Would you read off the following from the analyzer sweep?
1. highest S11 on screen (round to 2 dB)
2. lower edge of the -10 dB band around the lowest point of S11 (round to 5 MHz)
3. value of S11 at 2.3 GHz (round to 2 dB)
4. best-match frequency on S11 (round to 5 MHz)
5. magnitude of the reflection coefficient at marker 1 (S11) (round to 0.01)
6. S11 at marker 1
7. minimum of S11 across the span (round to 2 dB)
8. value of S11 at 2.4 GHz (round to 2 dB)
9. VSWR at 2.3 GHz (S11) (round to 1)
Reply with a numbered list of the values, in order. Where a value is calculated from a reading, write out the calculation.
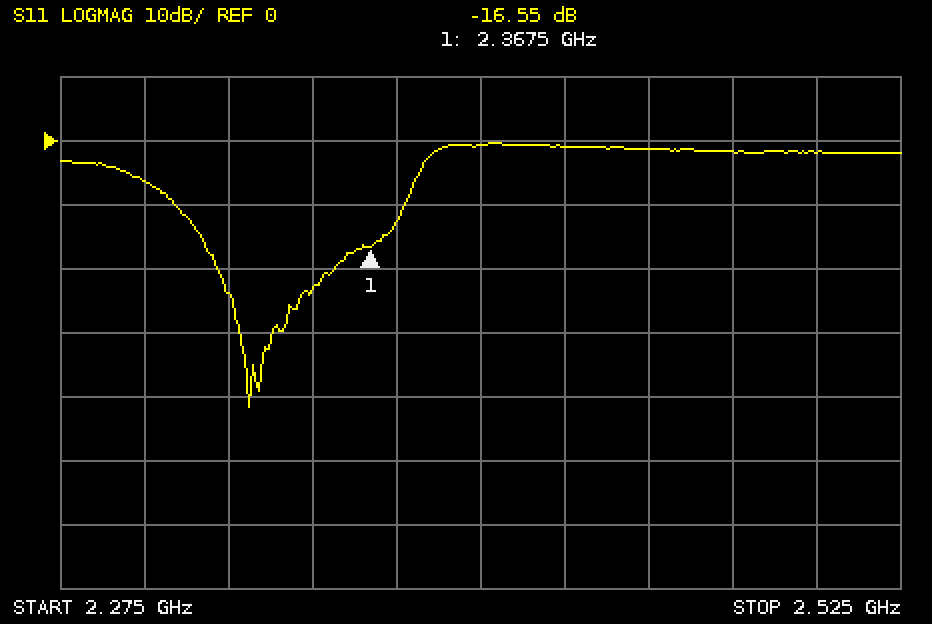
1. 0 dB
2. 2.310 GHz
3. -6 dB
4. 2.330 GHz
5. 10^(-16.55/20) ≈ 0.15
6. -16.55 dB
7. -42 dB
8. 0 dB
9. |Γ| = 10^(-6/20) = 0.5012; VSWR = (1 + 0.5012)/(1 − 0.5012) ≈ 3
